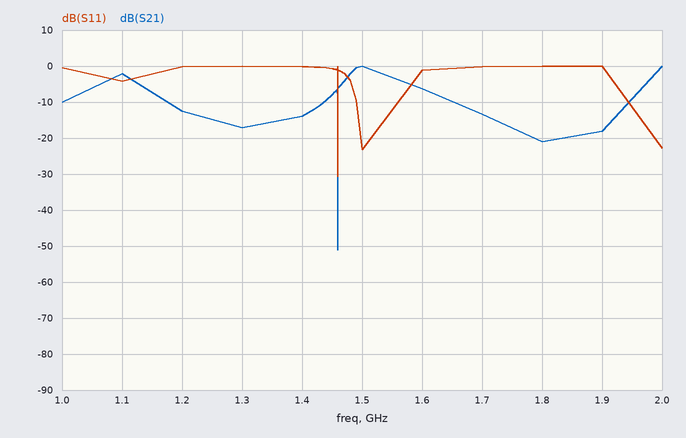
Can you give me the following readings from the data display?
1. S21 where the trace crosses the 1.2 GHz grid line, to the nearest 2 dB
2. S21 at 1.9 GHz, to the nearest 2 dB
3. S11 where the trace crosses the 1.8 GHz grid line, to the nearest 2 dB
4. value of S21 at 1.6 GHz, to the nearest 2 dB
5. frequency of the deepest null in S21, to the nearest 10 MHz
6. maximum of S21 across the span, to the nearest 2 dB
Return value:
-12 dB
-18 dB
0 dB
-6 dB
1.46 GHz
0 dB
